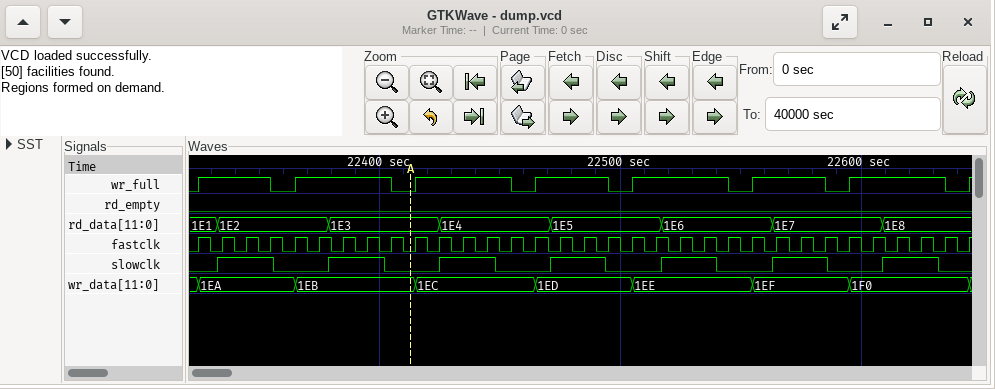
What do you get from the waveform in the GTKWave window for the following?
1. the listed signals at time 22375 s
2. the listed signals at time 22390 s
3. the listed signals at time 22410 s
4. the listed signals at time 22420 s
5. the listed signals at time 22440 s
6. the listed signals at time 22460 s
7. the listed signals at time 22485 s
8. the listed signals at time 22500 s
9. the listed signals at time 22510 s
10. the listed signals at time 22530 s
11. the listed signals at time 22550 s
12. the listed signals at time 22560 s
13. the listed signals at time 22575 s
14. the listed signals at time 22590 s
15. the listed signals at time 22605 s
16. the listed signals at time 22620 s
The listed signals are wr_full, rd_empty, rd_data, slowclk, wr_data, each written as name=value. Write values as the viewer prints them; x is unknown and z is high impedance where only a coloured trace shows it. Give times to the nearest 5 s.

wr_full=1, rd_empty=0, rd_data=1E2, slowclk=0, wr_data=1EB
wr_full=1, rd_empty=0, rd_data=1E3, slowclk=1, wr_data=1EB
wr_full=0, rd_empty=0, rd_data=1E3, slowclk=0, wr_data=1EB
wr_full=1, rd_empty=0, rd_data=1E3, slowclk=0, wr_data=1EC
wr_full=1, rd_empty=0, rd_data=1E4, slowclk=1, wr_data=1EC
wr_full=0, rd_empty=0, rd_data=1E4, slowclk=0, wr_data=1EC
wr_full=1, rd_empty=0, rd_data=1E5, slowclk=1, wr_data=1ED
wr_full=0, rd_empty=0, rd_data=1E5, slowclk=0, wr_data=1ED
wr_full=1, rd_empty=0, rd_data=1E5, slowclk=0, wr_data=1EE
wr_full=1, rd_empty=0, rd_data=1E6, slowclk=1, wr_data=1EE
wr_full=0, rd_empty=0, rd_data=1E6, slowclk=0, wr_data=1EE
wr_full=1, rd_empty=0, rd_data=1E6, slowclk=0, wr_data=1EF
wr_full=1, rd_empty=0, rd_data=1E7, slowclk=1, wr_data=1EF
wr_full=0, rd_empty=0, rd_data=1E7, slowclk=0, wr_data=1EF
wr_full=1, rd_empty=0, rd_data=1E7, slowclk=0, wr_data=1F0
wr_full=1, rd_empty=0, rd_data=1E8, slowclk=1, wr_data=1F0
